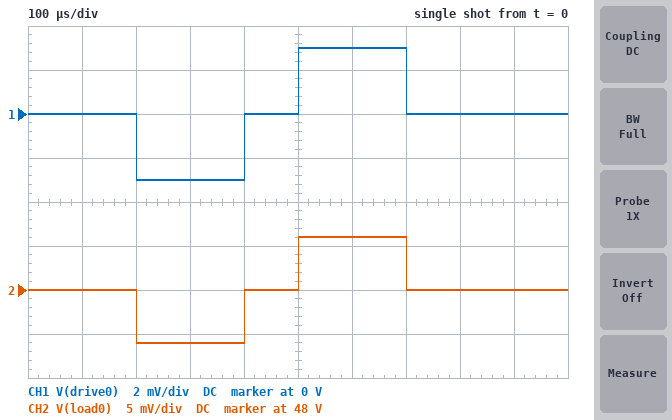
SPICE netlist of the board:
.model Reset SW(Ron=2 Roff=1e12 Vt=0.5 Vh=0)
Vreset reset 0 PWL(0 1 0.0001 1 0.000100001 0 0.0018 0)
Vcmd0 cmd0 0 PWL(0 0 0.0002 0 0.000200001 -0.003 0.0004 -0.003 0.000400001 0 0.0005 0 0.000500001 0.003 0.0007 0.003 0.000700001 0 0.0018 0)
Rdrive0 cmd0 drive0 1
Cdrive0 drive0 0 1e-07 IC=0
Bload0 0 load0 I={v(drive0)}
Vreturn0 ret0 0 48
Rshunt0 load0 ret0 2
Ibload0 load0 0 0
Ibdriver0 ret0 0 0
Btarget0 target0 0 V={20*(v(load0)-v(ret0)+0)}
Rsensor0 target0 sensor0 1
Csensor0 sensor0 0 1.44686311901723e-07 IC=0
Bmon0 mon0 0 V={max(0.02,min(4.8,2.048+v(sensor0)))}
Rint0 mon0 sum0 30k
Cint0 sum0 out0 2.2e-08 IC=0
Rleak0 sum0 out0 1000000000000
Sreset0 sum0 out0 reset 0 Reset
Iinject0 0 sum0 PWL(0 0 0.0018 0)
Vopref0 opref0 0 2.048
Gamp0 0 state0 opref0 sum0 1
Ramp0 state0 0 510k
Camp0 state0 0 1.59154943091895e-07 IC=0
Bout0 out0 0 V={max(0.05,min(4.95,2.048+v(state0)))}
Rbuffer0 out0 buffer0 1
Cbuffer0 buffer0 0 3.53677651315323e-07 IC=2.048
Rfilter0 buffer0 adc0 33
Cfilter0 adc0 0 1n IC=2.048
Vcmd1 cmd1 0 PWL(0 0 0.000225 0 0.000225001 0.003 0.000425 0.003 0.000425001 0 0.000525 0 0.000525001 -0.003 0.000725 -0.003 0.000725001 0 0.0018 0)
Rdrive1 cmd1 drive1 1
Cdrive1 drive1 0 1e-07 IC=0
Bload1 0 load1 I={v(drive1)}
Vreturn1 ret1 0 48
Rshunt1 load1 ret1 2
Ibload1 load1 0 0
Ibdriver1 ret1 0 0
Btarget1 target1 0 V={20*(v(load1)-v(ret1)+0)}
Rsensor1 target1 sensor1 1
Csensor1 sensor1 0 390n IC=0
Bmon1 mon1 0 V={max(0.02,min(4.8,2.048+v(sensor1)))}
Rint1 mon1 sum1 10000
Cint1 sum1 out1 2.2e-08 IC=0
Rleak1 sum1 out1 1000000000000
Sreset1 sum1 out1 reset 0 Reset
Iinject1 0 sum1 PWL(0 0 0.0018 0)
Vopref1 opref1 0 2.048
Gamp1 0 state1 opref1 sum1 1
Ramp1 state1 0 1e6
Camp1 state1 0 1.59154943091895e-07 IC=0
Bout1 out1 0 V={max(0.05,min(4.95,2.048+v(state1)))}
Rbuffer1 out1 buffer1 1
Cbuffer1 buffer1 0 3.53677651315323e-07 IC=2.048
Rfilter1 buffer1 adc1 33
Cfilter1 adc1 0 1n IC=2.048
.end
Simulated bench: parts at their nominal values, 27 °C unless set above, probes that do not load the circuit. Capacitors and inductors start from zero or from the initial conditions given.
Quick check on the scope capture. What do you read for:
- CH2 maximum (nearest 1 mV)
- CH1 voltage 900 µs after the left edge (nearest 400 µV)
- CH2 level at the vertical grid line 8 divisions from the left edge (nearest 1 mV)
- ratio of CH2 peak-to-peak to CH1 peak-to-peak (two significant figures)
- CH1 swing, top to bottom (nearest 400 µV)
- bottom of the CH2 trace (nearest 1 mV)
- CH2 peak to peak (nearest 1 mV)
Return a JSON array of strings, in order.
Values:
["48.006 V", "0 V", "48.000 V", "2.0", "6.0 mV", "47.994 V", "12 mV"]
